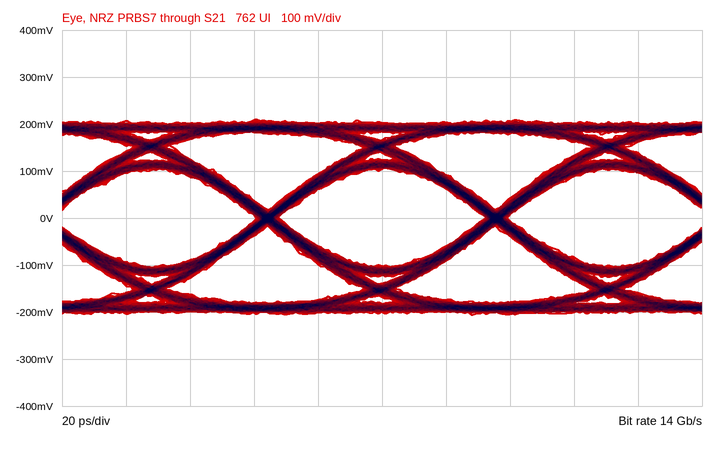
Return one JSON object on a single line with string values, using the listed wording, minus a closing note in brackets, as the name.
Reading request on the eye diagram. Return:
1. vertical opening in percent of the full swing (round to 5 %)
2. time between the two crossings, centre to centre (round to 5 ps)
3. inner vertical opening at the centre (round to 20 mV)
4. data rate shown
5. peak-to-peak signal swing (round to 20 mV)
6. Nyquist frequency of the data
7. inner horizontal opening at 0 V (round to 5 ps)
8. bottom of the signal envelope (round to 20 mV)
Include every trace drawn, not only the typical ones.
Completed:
{"vertical opening in percent of the full swing": "50 %", "time between the two crossings, centre to centre": "70 ps", "inner vertical opening at the centre": "200 mV", "data rate shown": "14 Gb/s", "peak-to-peak signal swing": "420 mV", "Nyquist frequency of the data": "7 GHz", "inner horizontal opening at 0 V": "65 ps", "bottom of the signal envelope": "-200 mV"}
